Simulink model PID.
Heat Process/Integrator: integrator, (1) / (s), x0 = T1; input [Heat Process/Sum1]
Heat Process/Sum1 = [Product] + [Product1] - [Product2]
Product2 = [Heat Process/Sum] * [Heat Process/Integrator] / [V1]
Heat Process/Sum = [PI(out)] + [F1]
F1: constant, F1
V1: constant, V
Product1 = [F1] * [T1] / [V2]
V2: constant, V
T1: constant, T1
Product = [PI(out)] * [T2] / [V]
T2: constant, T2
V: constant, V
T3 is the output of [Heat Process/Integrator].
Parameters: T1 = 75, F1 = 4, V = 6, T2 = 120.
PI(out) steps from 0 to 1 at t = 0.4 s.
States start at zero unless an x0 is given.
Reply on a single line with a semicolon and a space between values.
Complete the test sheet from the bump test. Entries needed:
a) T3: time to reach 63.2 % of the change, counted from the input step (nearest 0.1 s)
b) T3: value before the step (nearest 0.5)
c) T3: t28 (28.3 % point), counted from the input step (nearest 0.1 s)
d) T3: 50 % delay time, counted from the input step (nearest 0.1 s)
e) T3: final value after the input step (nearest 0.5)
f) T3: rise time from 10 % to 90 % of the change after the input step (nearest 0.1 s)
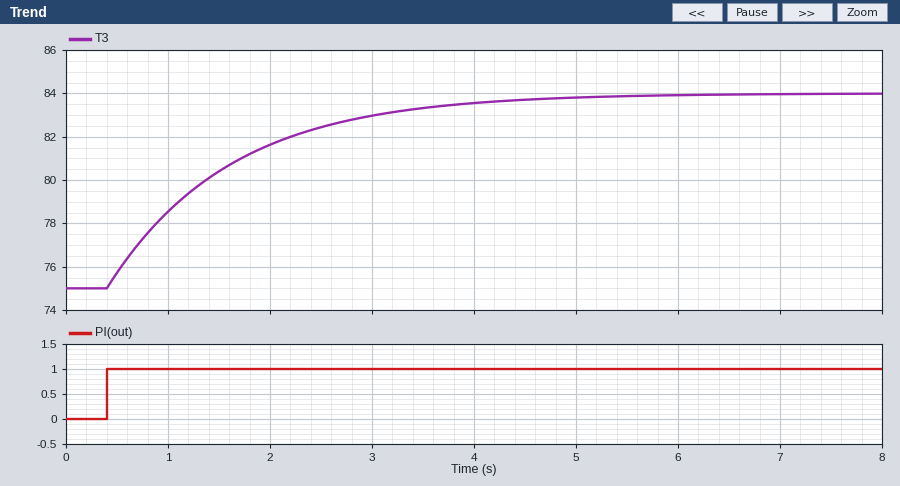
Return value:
1.2 s; 75.0; 0.4 s; 0.8 s; 84.0; 2.6 s
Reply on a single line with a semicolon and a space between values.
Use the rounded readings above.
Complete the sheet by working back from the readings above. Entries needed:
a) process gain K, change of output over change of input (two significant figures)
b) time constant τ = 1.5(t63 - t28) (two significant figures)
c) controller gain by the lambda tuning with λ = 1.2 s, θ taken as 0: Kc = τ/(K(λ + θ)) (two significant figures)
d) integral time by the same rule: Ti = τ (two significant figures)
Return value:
9.0; 1.2 s; 0.11; 1.2 s
